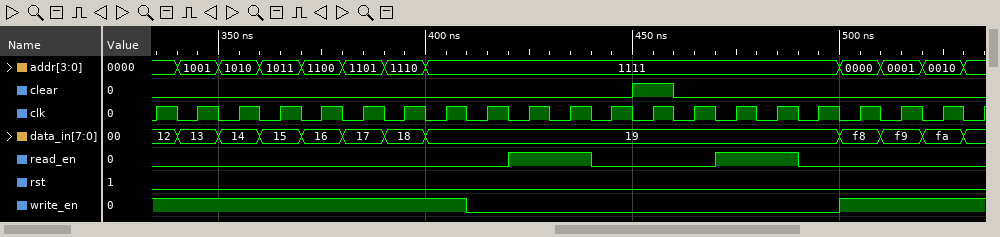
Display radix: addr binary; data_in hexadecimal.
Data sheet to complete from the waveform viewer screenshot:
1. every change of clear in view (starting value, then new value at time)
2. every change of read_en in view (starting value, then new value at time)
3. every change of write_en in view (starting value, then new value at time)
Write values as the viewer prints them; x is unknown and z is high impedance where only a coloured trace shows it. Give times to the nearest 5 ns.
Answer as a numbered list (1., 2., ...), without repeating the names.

1. 0, 1 at 450 ns, 0 at 460 ns
2. 0, 1 at 420 ns, 0 at 440 ns, 1 at 470 ns, 0 at 490 ns
3. 1, 0 at 410 ns, 1 at 500 ns
